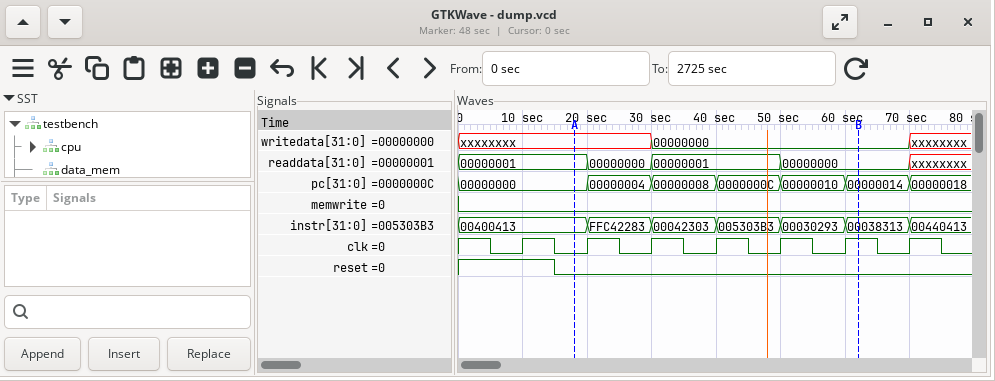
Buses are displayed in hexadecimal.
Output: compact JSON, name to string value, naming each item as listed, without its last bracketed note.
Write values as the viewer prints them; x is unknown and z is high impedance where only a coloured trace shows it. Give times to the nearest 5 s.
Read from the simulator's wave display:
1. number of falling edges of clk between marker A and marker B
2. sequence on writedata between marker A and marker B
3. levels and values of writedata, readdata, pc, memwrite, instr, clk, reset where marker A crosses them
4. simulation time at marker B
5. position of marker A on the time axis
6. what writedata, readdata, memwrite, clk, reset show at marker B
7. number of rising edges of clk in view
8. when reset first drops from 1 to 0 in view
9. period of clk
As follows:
{"number of falling edges of clk between marker A and marker B": "4", "sequence on writedata between marker A and marker B": "xxxxxxxx, 00000000", "levels and values of writedata, readdata, pc, memwrite, instr, clk, reset where marker A crosses them": "writedata=xxxxxxxx, readdata=00000001, pc=00000000, memwrite=0, instr=00400413, clk=0, reset=0", "simulation time at marker B": "60 s", "position of marker A on the time axis": "20 s", "what writedata, readdata, memwrite, clk, reset show at marker B": "writedata=00000000, readdata=00000000, memwrite=0, clk=1, reset=0", "number of rising edges of clk in view": "7", "when reset first drops from 1 to 0 in view": "15 s", "period of clk": "10 s"}
